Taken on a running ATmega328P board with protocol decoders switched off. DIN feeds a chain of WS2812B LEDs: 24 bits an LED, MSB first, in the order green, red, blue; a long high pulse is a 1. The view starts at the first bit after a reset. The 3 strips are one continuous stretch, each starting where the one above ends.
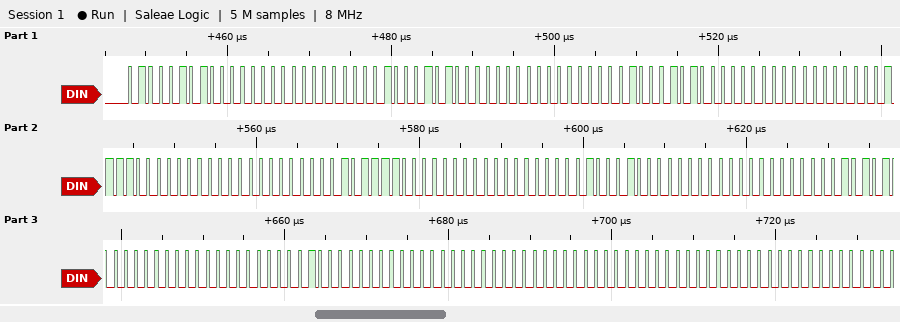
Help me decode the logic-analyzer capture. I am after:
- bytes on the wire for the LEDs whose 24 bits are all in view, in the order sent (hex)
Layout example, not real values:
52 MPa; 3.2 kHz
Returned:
45 00 00 45 00 00 45 00 00 3C 00 00 2F 00 00 22 00 00 15 00 00 08 00 00 00 00 00
